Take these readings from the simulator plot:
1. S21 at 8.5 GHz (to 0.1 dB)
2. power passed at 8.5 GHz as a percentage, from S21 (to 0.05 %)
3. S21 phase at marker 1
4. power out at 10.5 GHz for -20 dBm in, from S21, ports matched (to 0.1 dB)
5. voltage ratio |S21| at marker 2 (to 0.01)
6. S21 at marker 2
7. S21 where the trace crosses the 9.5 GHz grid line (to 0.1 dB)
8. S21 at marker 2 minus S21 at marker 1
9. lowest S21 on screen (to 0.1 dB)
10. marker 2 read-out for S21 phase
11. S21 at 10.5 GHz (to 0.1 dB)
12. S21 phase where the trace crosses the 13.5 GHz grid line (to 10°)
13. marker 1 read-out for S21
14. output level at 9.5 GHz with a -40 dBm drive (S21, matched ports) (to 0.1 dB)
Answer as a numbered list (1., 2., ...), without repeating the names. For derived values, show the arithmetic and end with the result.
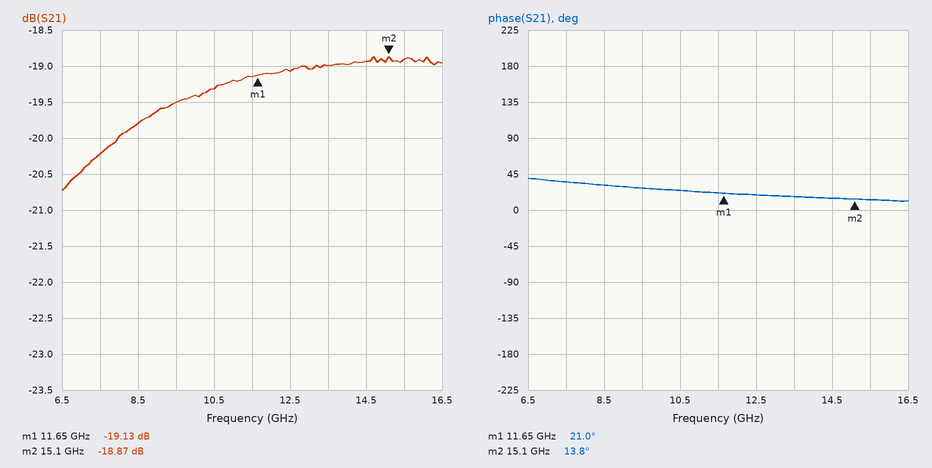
1. -19.8 dB
2. 10^(-19.8/10) ≈ 1.05 %
3. 21.0°
4. -20 dBm + (-19.3 dB) = -39.3 dBm
5. 10^(-18.87/20) ≈ 0.11
6. -18.87 dB
7. -19.5 dB
8. -18.87 − (-19.13) = 0.26 dB
9. -20.7 dB
10. 13.8°
11. -19.3 dB
12. 20°
13. -19.13 dB
14. -40 dBm + (-19.5 dB) = -59.5 dBm
